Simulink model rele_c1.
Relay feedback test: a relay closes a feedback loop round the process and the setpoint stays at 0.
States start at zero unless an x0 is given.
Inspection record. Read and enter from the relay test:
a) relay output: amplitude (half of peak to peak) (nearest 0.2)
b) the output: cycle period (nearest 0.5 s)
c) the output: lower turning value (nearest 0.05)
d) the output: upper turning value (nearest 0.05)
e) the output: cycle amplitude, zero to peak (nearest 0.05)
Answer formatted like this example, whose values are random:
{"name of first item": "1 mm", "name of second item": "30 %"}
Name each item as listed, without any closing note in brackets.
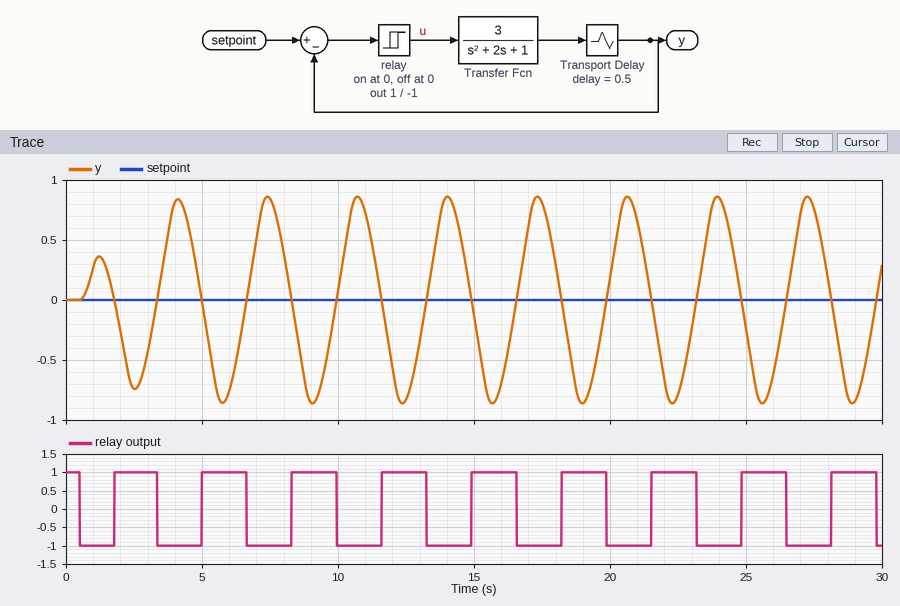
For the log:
{"relay output: amplitude (half of peak to peak)": "1.0", "the output: cycle period": "3.5 s", "the output: lower turning value": "-0.85", "the output: upper turning value": "0.85", "the output: cycle amplitude, zero to peak": "0.85"}
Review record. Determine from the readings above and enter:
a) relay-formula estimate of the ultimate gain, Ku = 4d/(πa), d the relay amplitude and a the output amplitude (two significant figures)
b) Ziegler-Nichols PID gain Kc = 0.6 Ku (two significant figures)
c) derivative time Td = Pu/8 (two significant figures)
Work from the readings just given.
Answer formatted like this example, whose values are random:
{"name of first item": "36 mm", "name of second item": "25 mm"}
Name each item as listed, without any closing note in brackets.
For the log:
{"relay-formula estimate of the ultimate gain, Ku = 4d/(πa), d the relay amplitude and a the output amplitude": "1.5", "Ziegler-Nichols PID gain Kc = 0.6 Ku": "0.90", "derivative time Td = Pu/8": "0.44 s"}
